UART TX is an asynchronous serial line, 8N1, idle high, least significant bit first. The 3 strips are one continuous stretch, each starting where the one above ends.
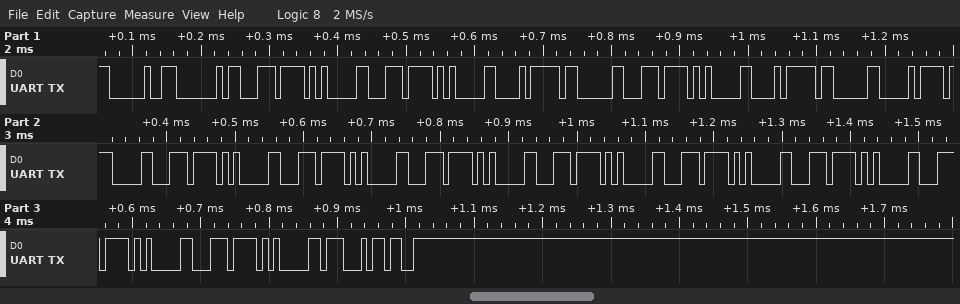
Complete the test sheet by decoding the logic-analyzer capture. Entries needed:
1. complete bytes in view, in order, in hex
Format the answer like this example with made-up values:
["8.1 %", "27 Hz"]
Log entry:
["20 40 DC 05 DC 05 E8 03 DC 05 E8 03 D0 07 DC 05 DC 05 DC 05 DC 05 DC 05 DC 05 DC 05 DC 05 47 F3"]
